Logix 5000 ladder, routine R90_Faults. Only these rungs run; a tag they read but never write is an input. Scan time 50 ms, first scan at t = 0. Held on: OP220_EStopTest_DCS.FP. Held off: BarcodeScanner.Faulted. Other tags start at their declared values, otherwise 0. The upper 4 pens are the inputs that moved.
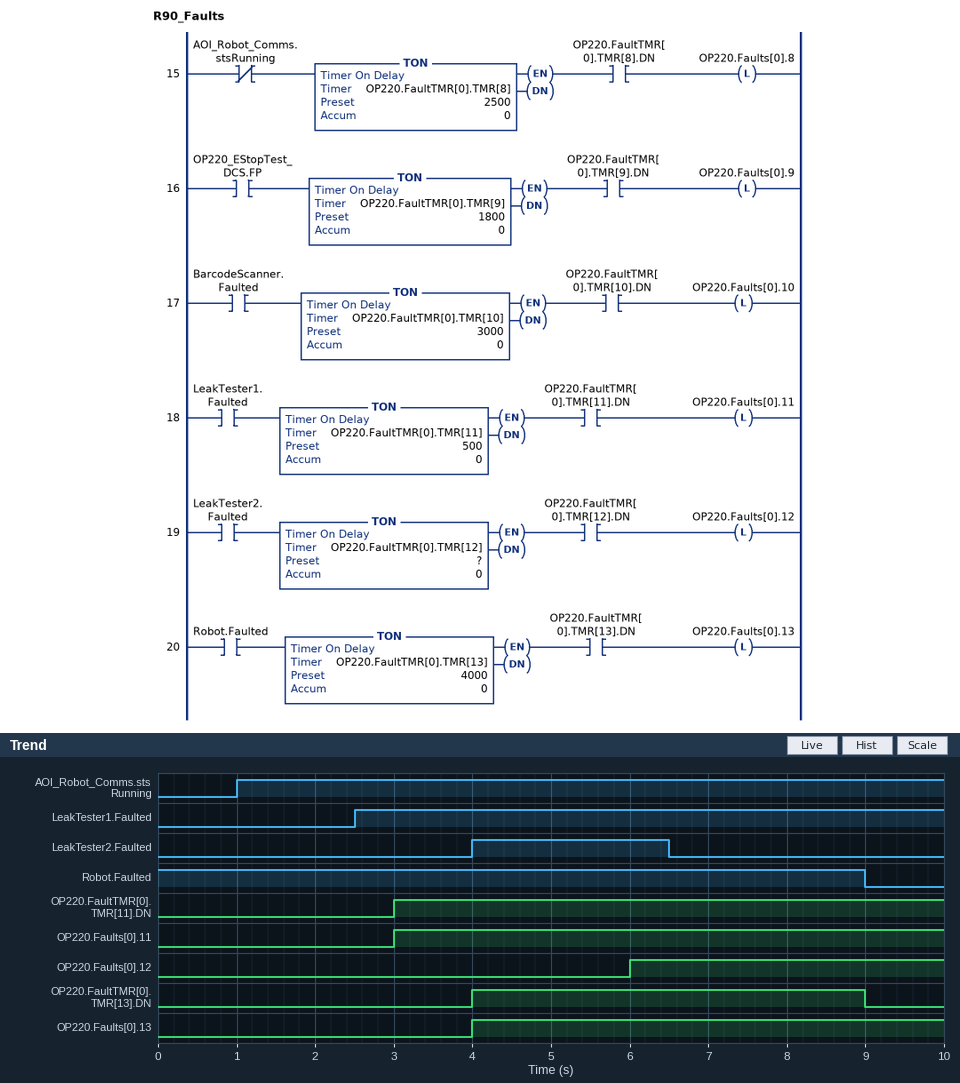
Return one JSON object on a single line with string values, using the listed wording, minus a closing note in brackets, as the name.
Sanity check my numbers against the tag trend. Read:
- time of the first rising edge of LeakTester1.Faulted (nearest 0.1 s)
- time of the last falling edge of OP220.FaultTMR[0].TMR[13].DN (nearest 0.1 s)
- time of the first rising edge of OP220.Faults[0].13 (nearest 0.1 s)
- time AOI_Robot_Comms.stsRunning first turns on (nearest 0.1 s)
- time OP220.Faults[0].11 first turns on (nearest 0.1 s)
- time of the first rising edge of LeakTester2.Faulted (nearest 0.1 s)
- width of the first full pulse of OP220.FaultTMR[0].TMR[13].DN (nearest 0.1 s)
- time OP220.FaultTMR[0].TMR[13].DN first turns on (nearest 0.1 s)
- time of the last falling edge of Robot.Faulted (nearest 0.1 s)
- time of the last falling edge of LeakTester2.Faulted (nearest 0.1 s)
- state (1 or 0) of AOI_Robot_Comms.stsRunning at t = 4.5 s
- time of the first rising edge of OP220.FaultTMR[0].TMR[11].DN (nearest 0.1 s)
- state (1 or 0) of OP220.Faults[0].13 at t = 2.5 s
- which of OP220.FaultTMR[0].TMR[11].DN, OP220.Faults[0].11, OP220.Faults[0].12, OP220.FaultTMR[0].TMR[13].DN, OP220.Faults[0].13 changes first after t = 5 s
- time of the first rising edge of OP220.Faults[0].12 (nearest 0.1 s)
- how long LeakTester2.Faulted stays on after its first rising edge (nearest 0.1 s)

{"time of the first rising edge of LeakTester1.Faulted": "2.5 s", "time of the last falling edge of OP220.FaultTMR[0].TMR[13].DN": "9.0 s", "time of the first rising edge of OP220.Faults[0].13": "4.0 s", "time AOI_Robot_Comms.stsRunning first turns on": "1.0 s", "time OP220.Faults[0].11 first turns on": "3.0 s", "time of the first rising edge of LeakTester2.Faulted": "4.0 s", "width of the first full pulse of OP220.FaultTMR[0].TMR[13].DN": "5.0 s", "time OP220.FaultTMR[0].TMR[13].DN first turns on": "4.0 s", "time of the last falling edge of Robot.Faulted": "9.0 s", "time of the last falling edge of LeakTester2.Faulted": "6.5 s", "state (1 or 0) of AOI_Robot_Comms.stsRunning at t = 4.5 s": "1", "time of the first rising edge of OP220.FaultTMR[0].TMR[11].DN": "3.0 s", "state (1 or 0) of OP220.Faults[0].13 at t = 2.5 s": "0", "which of OP220.FaultTMR[0].TMR[11].DN, OP220.Faults[0].11, OP220.Faults[0].12, OP220.FaultTMR[0].TMR[13].DN, OP220.Faults[0].13 changes first after t = 5 s": "OP220.Faults[0].12", "time of the first rising edge of OP220.Faults[0].12": "6.0 s", "how long LeakTester2.Faulted stays on after its first rising edge": "2.5 s"}
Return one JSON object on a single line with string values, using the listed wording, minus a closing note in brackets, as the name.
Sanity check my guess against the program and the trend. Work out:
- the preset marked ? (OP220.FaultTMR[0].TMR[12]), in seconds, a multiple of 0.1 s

{"the preset marked ? (OP220.FaultTMR[0].TMR[12]), in seconds, a multiple of 0.1 s": "2.0 s"}
